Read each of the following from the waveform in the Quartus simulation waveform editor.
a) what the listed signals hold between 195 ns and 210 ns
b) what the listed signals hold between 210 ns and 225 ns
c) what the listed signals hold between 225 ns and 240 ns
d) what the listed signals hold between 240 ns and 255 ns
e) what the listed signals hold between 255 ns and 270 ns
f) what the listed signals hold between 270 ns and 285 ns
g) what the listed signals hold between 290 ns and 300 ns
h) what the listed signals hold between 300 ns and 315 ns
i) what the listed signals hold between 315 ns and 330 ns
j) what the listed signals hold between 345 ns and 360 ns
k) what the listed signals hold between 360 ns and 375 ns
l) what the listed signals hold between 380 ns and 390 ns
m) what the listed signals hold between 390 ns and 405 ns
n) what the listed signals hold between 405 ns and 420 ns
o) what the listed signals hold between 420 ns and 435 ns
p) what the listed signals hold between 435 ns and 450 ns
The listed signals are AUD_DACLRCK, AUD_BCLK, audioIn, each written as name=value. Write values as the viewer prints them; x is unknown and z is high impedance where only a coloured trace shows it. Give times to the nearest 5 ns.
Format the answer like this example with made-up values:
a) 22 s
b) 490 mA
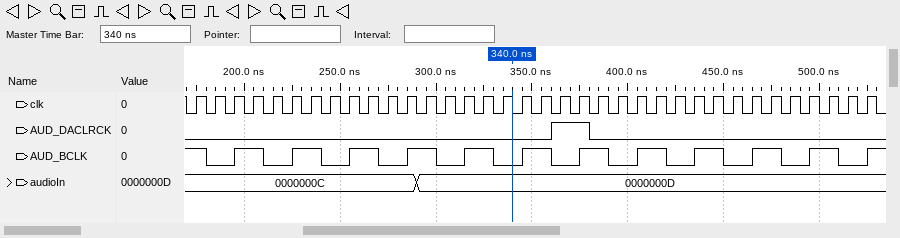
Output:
a) AUD_DACLRCK=0, AUD_BCLK=1, audioIn=0000000C
b) AUD_DACLRCK=0, AUD_BCLK=0, audioIn=0000000C
c) AUD_DACLRCK=0, AUD_BCLK=1, audioIn=0000000C
d) AUD_DACLRCK=0, AUD_BCLK=0, audioIn=0000000C
e) AUD_DACLRCK=0, AUD_BCLK=1, audioIn=0000000C
f) AUD_DACLRCK=0, AUD_BCLK=0, audioIn=0000000C
g) AUD_DACLRCK=0, AUD_BCLK=1, audioIn=0000000D
h) AUD_DACLRCK=0, AUD_BCLK=0, audioIn=0000000D
i) AUD_DACLRCK=0, AUD_BCLK=1, audioIn=0000000D
j) AUD_DACLRCK=0, AUD_BCLK=1, audioIn=0000000D
k) AUD_DACLRCK=1, AUD_BCLK=0, audioIn=0000000D
l) AUD_DACLRCK=0, AUD_BCLK=1, audioIn=0000000D
m) AUD_DACLRCK=0, AUD_BCLK=0, audioIn=0000000D
n) AUD_DACLRCK=0, AUD_BCLK=1, audioIn=0000000D
o) AUD_DACLRCK=0, AUD_BCLK=0, audioIn=0000000D
p) AUD_DACLRCK=0, AUD_BCLK=1, audioIn=0000000D
